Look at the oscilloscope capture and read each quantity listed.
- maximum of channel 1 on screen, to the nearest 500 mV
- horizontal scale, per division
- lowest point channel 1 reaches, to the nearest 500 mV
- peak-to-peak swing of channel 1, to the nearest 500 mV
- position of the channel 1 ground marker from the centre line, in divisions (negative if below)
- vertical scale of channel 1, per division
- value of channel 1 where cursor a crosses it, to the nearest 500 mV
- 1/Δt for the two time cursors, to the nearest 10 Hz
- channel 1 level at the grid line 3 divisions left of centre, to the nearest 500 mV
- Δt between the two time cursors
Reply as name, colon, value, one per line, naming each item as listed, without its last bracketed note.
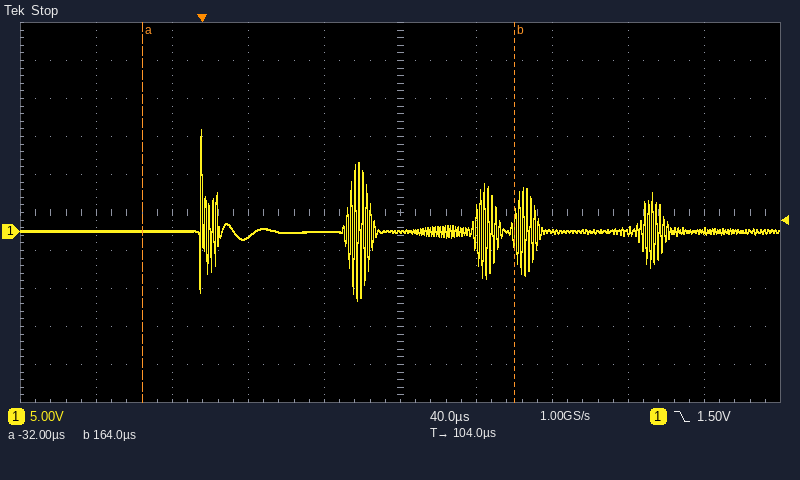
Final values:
maximum of channel 1 on screen, to the nearest 500 mV: 13.5 V
horizontal scale, per division: 40 µs
lowest point channel 1 reaches, to the nearest 500 mV: -9.0 V
peak-to-peak swing of channel 1, to the nearest 500 mV: 22.5 V
position of the channel 1 ground marker from the centre line, in divisions: -0.5 div
vertical scale of channel 1, per division: 5 V
value of channel 1 where cursor a crosses it, to the nearest 500 mV: 0.0 V
1/Δt for the two time cursors, to the nearest 10 Hz: 5.10 kHz
channel 1 level at the grid line 3 divisions left of centre, to the nearest 500 mV: 0.0 V
Δt between the two time cursors: 196 µs
